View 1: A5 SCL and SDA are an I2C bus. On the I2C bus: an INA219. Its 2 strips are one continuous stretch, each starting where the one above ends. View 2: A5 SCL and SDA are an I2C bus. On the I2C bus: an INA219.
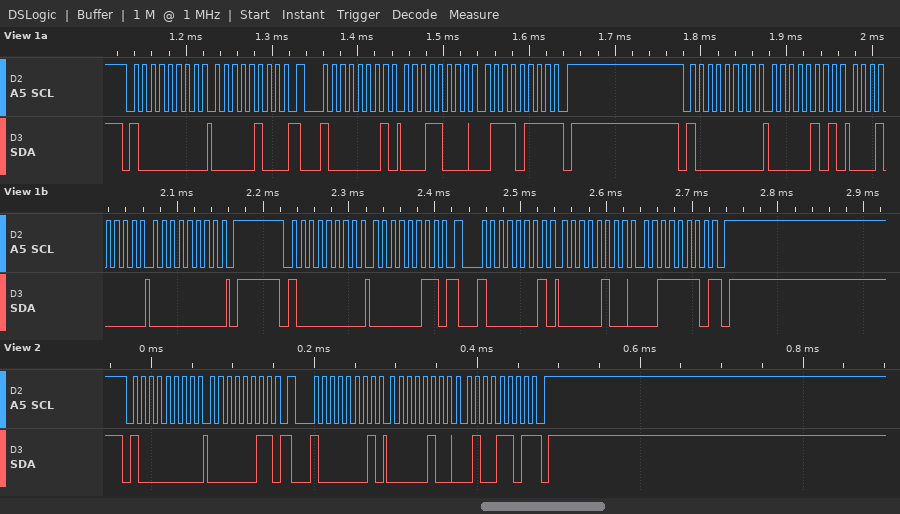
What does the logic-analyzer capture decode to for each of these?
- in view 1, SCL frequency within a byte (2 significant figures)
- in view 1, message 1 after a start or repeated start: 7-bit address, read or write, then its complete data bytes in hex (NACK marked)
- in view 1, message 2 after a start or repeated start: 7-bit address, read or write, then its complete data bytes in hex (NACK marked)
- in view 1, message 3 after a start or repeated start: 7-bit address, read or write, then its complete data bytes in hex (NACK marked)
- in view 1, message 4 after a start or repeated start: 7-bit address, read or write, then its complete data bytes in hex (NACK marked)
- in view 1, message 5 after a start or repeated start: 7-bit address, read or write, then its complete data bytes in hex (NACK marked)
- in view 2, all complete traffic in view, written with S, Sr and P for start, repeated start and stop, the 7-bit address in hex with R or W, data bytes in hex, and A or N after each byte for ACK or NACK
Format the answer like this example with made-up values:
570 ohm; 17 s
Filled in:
100 kHz; 0x40 write: 04; 0x40 read: 18 77 NACK; 0x40 write: 05 10 00; 0x40 write: 03; 0x40 read: 04 3E NACK; S 40W A 03 A Sr 40R A 04 A 4D N P
